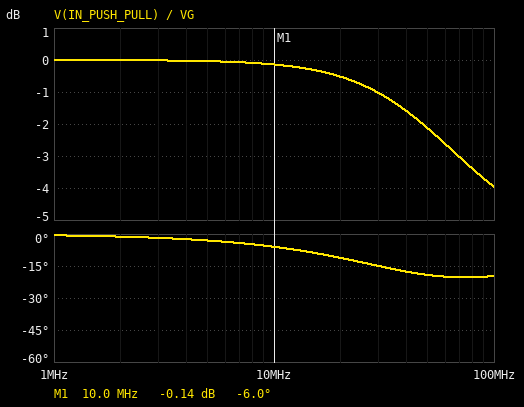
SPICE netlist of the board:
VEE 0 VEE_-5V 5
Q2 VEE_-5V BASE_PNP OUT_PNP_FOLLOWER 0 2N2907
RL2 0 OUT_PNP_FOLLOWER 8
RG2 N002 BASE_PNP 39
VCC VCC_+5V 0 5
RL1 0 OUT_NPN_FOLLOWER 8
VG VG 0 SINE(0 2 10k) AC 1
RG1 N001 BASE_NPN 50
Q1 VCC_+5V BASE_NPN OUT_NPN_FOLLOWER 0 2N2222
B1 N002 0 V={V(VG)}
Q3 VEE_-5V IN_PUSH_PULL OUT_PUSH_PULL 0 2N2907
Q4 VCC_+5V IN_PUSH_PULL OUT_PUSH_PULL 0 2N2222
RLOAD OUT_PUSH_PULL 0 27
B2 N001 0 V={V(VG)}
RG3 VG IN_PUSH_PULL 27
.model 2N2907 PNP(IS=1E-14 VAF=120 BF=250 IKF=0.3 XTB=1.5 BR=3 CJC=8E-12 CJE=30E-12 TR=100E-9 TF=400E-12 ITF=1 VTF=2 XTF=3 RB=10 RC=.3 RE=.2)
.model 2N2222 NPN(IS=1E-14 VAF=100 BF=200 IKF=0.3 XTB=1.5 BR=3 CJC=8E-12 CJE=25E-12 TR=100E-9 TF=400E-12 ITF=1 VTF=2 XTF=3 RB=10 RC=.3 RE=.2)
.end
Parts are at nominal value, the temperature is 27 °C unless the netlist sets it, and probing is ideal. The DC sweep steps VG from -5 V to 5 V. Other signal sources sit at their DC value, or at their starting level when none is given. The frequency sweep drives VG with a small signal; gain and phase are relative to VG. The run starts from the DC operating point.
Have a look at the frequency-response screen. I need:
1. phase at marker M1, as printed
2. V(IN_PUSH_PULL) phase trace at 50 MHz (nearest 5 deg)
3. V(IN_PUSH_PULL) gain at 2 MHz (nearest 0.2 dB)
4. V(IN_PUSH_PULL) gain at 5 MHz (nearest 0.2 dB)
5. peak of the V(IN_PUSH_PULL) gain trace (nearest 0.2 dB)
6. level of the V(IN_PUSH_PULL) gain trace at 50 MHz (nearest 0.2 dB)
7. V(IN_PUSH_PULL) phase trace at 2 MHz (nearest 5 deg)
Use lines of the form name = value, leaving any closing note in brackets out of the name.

phase at marker M1, as printed = -6.0 deg
V(IN_PUSH_PULL) phase trace at 50 MHz = -20 deg
V(IN_PUSH_PULL) gain at 2 MHz = 0 dB
V(IN_PUSH_PULL) gain at 5 MHz = 0 dB
peak of the V(IN_PUSH_PULL) gain trace = 0 dB
level of the V(IN_PUSH_PULL) gain trace at 50 MHz = -2.2 dB
V(IN_PUSH_PULL) phase trace at 2 MHz = 0 deg
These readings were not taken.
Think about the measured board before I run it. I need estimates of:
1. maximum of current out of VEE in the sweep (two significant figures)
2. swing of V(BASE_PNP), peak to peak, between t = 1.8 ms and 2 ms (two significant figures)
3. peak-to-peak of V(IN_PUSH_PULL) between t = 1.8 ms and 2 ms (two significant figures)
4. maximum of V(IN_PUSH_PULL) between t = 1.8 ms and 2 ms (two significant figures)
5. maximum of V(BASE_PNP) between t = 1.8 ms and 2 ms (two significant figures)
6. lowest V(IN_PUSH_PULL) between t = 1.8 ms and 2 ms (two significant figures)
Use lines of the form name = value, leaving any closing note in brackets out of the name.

maximum of current out of VEE in the sweep = 630 mA
swing of V(BASE_PNP), peak to peak, between t = 1.8 ms and 2 ms = 4.0 V
peak-to-peak of V(IN_PUSH_PULL) between t = 1.8 ms and 2 ms = 4.0 V
maximum of V(IN_PUSH_PULL) between t = 1.8 ms and 2 ms = 2.0 V
maximum of V(BASE_PNP) between t = 1.8 ms and 2 ms = 2.0 V
lowest V(IN_PUSH_PULL) between t = 1.8 ms and 2 ms = -2.0 V
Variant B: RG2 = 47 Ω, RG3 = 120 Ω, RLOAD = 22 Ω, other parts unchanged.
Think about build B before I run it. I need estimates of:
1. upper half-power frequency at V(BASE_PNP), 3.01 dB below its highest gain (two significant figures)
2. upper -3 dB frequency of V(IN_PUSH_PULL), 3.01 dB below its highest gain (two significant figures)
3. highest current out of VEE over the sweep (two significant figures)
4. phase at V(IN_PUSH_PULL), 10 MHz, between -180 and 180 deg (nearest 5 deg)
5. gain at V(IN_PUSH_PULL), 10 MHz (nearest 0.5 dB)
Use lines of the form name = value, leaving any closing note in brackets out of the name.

upper half-power frequency at V(BASE_PNP), 3.01 dB below its highest gain = 79 MHz
upper -3 dB frequency of V(IN_PUSH_PULL), 3.01 dB below its highest gain = 18 MHz
highest current out of VEE over the sweep = 650 mA
phase at V(IN_PUSH_PULL), 10 MHz, between -180 and 180 deg = -25 deg
gain at V(IN_PUSH_PULL), 10 MHz = -1.0 dB
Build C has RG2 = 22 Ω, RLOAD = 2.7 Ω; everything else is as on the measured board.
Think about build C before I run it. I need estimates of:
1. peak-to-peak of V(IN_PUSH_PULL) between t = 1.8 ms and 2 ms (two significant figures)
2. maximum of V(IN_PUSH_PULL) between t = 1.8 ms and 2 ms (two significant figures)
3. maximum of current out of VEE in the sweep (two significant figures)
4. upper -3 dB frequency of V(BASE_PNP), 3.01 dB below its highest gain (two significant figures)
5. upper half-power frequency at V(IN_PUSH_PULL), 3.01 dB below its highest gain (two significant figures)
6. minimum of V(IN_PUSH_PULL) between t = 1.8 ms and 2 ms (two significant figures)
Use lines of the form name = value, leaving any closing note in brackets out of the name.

peak-to-peak of V(IN_PUSH_PULL) between t = 1.8 ms and 2 ms = 3.8 V
maximum of V(IN_PUSH_PULL) between t = 1.8 ms and 2 ms = 1.9 V
maximum of current out of VEE in the sweep = 1.6 A
upper -3 dB frequency of V(BASE_PNP), 3.01 dB below its highest gain = 150 MHz
upper half-power frequency at V(IN_PUSH_PULL), 3.01 dB below its highest gain = 77 MHz
minimum of V(IN_PUSH_PULL) between t = 1.8 ms and 2 ms = -1.9 V
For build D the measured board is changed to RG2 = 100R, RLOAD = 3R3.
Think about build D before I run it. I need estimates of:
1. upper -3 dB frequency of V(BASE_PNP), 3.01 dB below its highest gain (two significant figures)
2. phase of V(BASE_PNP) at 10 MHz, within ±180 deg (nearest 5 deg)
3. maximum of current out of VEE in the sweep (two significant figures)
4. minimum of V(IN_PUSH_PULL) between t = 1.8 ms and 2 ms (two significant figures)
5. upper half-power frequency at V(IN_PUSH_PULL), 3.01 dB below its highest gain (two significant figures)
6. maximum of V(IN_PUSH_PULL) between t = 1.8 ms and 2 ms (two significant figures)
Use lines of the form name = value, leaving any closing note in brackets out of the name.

upper -3 dB frequency of V(BASE_PNP), 3.01 dB below its highest gain = 41 MHz
phase of V(BASE_PNP) at 10 MHz, within ±180 deg = -10 deg
maximum of current out of VEE in the sweep = 1.4 A
minimum of V(IN_PUSH_PULL) between t = 1.8 ms and 2 ms = -1.9 V
upper half-power frequency at V(IN_PUSH_PULL), 3.01 dB below its highest gain = 77 MHz
maximum of V(IN_PUSH_PULL) between t = 1.8 ms and 2 ms = 1.9 V
